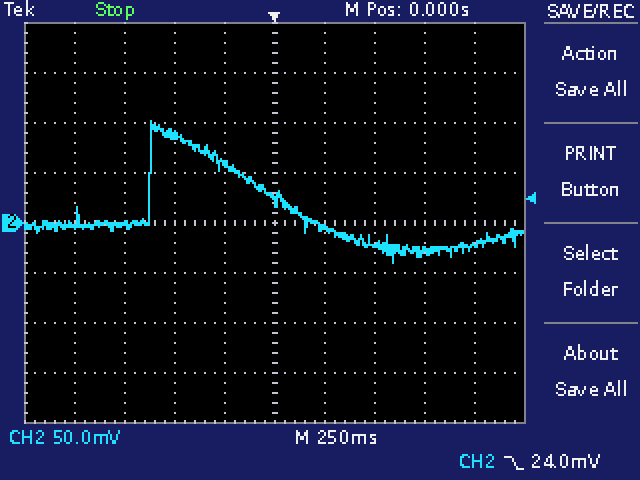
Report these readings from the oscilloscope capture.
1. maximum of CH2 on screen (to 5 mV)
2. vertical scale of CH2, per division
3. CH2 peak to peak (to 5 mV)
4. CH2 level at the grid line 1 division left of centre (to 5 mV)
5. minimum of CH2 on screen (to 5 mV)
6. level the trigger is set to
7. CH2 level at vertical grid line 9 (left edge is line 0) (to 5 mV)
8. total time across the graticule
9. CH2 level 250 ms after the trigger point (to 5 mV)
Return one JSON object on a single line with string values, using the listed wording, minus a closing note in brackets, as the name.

{"maximum of CH2 on screen": "100 mV", "vertical scale of CH2, per division": "50 mV", "CH2 peak to peak": "140 mV", "CH2 level at the grid line 1 division left of centre": "60 mV", "minimum of CH2 on screen": "-40 mV", "level the trigger is set to": "24.0 mV", "CH2 level at vertical grid line 9 (left edge is line 0)": "-20 mV", "total time across the graticule": "2.5 s", "CH2 level 250 ms after the trigger point": "-5 mV"}
